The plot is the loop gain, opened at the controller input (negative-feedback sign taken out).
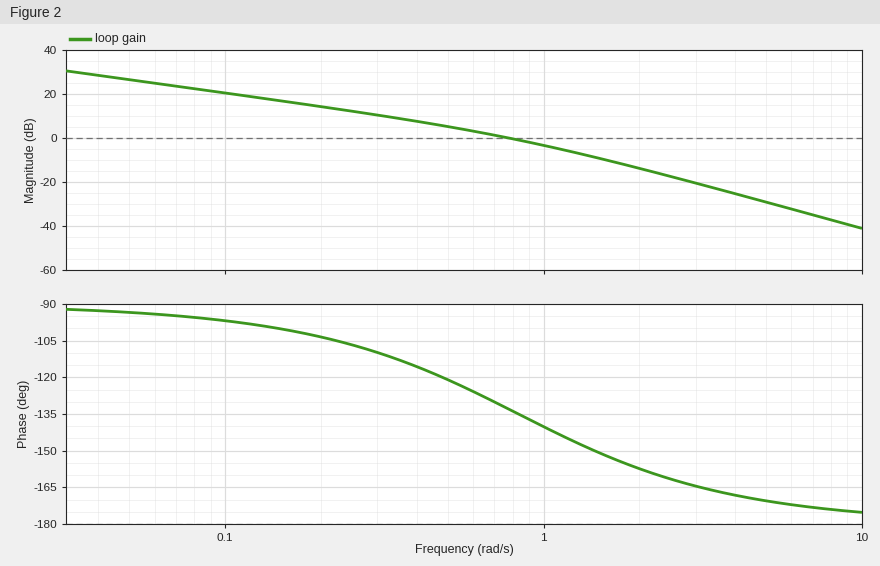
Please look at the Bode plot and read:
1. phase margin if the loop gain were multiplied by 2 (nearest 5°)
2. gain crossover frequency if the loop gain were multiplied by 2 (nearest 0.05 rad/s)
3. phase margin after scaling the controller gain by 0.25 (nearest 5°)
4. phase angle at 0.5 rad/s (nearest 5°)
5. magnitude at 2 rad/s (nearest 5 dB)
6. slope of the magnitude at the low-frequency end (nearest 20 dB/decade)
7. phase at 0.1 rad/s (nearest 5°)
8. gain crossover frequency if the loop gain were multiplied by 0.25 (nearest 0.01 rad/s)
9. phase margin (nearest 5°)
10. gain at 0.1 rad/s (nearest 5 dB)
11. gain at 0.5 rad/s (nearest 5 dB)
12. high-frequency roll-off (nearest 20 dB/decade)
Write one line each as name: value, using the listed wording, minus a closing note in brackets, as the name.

phase margin if the loop gain were multiplied by 2: 35°
gain crossover frequency if the loop gain were multiplied by 2: 1.20 rad/s
phase margin after scaling the controller gain by 0.25: 75°
phase angle at 0.5 rad/s: -120°
magnitude at 2 rad/s: -15 dB
slope of the magnitude at the low-frequency end: -20 dB/decade
phase at 0.1 rad/s: -95°
gain crossover frequency if the loop gain were multiplied by 0.25: 0.25 rad/s
phase margin: 45°
gain at 0.1 rad/s: 20 dB
gain at 0.5 rad/s: 5 dB
high-frequency roll-off: -40 dB/decade
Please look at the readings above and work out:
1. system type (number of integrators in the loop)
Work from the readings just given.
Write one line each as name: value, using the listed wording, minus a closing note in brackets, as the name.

system type: 1
